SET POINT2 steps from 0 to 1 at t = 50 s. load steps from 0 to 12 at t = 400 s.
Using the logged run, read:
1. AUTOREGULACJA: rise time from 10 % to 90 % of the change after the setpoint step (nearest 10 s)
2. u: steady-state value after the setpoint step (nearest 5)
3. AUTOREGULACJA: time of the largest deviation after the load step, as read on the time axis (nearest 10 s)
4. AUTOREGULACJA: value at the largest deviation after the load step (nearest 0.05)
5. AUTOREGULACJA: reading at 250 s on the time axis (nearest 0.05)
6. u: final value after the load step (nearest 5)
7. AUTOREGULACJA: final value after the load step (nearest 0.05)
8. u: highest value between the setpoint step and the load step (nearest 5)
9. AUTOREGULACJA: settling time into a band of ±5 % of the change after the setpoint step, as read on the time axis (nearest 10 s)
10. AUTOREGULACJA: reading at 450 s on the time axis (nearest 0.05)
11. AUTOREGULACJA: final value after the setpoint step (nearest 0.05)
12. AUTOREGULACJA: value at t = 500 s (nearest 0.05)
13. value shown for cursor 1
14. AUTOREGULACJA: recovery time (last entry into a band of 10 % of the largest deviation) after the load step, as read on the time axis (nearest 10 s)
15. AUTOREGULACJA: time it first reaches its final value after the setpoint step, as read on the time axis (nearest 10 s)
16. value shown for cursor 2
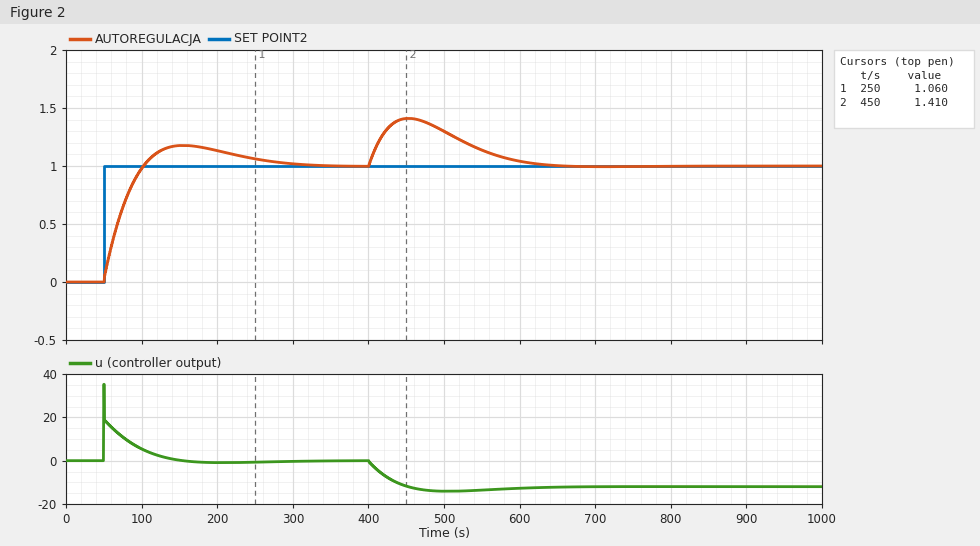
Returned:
40 s
0
450 s
1.40
1.05
-10
1.00
35
260 s
1.40
1.00
1.30
1.060
600 s
100 s
1.410
